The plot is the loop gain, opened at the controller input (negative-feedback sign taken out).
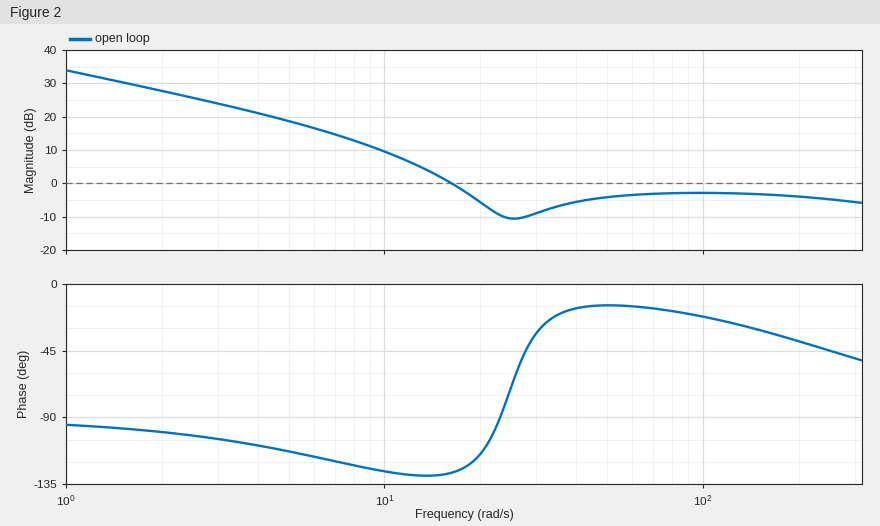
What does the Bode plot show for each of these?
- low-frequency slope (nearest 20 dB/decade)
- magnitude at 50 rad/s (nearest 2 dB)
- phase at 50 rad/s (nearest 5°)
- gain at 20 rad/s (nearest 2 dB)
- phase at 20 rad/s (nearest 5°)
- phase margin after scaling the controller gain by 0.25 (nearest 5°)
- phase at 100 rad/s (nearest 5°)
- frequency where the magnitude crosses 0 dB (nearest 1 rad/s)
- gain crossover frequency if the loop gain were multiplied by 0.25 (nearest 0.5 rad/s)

-20 dB/decade
-4 dB
-15°
-6 dB
-115°
55°
-20°
16 rad/s
8.5 rad/s
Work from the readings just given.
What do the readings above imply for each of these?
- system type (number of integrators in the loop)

1
